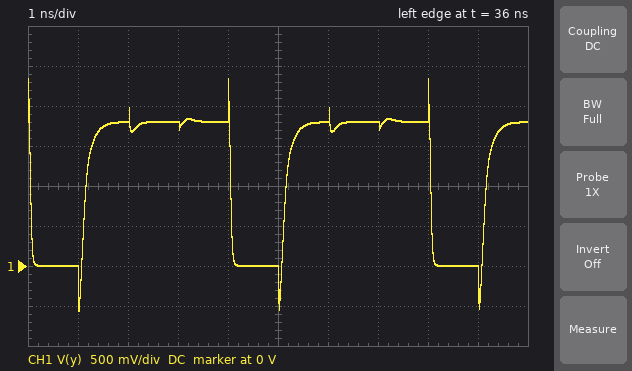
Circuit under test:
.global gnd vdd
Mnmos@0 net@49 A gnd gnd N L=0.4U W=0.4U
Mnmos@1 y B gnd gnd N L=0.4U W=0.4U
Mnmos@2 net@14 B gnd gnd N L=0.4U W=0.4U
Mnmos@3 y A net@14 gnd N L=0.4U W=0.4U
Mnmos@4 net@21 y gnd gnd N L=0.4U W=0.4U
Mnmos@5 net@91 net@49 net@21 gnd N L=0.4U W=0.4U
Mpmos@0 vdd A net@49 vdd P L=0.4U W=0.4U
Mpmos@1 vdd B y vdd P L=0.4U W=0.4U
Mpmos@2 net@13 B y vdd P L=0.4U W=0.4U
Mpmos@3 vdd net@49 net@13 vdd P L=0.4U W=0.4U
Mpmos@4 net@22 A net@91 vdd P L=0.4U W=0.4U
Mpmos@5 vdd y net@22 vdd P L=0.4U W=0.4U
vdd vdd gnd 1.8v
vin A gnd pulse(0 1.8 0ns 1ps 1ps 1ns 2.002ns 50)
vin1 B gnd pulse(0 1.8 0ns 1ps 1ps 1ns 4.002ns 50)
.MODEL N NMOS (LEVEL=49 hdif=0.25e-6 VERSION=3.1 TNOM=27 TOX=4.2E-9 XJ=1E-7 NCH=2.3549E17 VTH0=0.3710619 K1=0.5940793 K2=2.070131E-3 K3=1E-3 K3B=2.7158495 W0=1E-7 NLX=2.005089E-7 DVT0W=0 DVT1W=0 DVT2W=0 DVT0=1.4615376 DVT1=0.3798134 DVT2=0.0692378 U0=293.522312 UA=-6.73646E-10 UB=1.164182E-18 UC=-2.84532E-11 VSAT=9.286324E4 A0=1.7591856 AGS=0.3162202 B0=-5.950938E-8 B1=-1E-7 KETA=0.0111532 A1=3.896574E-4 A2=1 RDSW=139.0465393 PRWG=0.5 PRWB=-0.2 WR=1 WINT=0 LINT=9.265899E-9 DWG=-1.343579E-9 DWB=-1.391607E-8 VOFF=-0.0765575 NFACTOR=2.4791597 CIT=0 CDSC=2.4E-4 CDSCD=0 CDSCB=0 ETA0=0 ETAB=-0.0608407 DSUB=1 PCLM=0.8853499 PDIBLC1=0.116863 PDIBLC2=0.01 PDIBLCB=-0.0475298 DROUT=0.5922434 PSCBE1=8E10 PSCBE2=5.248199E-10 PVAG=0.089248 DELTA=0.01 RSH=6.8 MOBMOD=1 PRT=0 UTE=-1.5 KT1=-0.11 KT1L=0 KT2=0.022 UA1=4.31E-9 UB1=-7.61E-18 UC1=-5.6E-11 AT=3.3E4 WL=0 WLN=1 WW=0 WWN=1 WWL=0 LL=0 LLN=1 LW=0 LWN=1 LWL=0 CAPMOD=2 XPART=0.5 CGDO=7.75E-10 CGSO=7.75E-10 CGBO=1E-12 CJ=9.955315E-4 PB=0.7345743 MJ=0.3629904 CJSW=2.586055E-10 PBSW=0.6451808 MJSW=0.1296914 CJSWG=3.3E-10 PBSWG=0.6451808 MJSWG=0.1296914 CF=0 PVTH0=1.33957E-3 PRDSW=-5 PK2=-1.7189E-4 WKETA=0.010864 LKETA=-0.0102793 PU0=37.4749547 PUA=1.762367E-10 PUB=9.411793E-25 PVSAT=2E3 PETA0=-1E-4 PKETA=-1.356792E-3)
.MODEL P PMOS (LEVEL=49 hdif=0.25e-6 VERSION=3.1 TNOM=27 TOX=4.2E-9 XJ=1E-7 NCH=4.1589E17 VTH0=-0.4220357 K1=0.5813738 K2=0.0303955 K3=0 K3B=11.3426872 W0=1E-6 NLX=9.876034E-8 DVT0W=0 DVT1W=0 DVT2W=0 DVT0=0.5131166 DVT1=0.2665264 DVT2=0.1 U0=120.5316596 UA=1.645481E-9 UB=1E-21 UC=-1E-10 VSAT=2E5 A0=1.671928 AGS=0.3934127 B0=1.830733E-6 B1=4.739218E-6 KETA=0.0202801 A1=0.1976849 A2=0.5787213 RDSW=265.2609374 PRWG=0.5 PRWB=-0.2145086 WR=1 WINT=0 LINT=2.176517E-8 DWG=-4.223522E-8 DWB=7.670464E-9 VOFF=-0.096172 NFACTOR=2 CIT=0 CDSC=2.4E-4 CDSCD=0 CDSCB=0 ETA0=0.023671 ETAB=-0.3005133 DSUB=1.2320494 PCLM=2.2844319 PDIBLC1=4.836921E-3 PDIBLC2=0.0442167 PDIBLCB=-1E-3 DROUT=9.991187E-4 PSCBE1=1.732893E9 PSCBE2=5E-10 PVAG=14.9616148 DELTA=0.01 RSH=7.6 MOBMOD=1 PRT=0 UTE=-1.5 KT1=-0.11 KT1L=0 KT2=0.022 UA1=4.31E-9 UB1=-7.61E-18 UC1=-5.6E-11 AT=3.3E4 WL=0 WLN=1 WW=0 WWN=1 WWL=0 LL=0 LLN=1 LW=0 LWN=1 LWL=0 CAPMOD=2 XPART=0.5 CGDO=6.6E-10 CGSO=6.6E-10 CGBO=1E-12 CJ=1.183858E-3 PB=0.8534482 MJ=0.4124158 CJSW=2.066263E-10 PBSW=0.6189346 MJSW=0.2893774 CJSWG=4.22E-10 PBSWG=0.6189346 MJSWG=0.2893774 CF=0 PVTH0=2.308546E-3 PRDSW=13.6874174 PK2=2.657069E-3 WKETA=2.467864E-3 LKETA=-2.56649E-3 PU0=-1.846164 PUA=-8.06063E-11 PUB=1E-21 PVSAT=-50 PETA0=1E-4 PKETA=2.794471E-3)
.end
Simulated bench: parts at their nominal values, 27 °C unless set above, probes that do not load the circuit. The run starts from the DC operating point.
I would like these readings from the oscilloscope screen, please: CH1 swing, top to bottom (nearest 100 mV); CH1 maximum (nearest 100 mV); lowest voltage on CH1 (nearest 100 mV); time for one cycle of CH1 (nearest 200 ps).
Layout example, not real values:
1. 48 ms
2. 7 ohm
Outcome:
1. 2.9 V
2. 2.3 V
3. -600 mV
4. 4.0 ns
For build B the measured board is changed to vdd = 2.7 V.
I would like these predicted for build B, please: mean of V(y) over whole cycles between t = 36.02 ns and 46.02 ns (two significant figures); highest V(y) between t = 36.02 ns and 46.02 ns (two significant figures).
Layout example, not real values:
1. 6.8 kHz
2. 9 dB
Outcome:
1. 2.0 V
2. 3.3 V
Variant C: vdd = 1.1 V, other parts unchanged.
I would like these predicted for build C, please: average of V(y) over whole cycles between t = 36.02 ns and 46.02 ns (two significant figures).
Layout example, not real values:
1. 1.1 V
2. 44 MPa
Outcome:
1. 670 mV
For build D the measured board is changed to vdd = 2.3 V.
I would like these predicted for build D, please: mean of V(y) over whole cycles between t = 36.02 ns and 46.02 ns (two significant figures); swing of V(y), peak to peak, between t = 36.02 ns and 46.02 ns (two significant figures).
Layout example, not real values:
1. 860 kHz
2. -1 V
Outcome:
1. 1.7 V
2. 3.4 V
